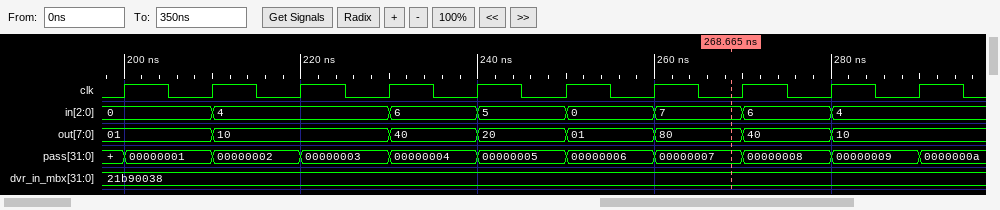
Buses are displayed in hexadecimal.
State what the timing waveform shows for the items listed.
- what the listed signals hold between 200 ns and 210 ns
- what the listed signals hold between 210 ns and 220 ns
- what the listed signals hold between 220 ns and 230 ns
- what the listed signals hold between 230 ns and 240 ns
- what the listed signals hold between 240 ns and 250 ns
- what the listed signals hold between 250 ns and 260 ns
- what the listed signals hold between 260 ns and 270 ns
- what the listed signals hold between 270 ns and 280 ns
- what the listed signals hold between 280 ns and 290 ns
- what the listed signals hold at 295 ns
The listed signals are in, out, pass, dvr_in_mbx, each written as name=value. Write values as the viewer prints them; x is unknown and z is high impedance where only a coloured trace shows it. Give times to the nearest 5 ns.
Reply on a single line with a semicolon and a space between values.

in=0, out=01, pass=00000001, dvr_in_mbx=21b90038; in=4, out=10, pass=00000002, dvr_in_mbx=21b90038; in=4, out=10, pass=00000003, dvr_in_mbx=21b90038; in=6, out=40, pass=00000004, dvr_in_mbx=21b90038; in=5, out=20, pass=00000005, dvr_in_mbx=21b90038; in=0, out=01, pass=00000006, dvr_in_mbx=21b90038; in=7, out=80, pass=00000007, dvr_in_mbx=21b90038; in=6, out=40, pass=00000008, dvr_in_mbx=21b90038; in=4, out=10, pass=00000009, dvr_in_mbx=21b90038; in=4, out=10, pass=0000000a, dvr_in_mbx=21b90038
